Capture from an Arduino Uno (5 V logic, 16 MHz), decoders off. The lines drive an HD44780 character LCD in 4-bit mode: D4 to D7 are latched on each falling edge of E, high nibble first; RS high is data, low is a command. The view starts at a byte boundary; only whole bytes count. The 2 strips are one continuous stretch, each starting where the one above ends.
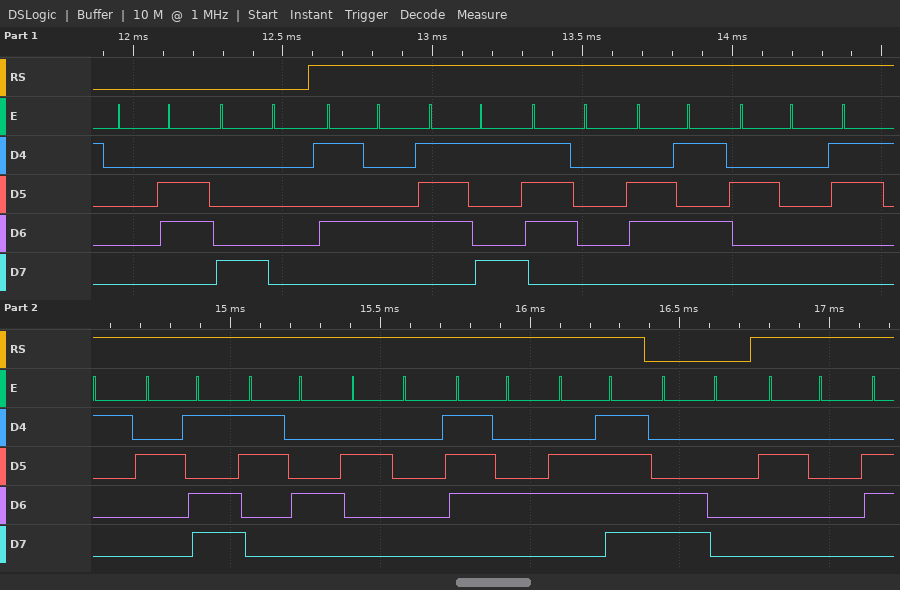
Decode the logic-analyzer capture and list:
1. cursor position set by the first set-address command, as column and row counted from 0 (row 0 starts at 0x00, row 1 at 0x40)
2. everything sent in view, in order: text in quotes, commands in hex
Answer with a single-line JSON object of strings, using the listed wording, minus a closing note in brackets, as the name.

{"cursor position set by the first set-address command, as column and row counted from 0": "column 0, row 0", "everything sent in view, in order: text in quotes, commands in hex": "0x06 0x80 \"Type 1-4 to\" 0xC0 \" \""}
